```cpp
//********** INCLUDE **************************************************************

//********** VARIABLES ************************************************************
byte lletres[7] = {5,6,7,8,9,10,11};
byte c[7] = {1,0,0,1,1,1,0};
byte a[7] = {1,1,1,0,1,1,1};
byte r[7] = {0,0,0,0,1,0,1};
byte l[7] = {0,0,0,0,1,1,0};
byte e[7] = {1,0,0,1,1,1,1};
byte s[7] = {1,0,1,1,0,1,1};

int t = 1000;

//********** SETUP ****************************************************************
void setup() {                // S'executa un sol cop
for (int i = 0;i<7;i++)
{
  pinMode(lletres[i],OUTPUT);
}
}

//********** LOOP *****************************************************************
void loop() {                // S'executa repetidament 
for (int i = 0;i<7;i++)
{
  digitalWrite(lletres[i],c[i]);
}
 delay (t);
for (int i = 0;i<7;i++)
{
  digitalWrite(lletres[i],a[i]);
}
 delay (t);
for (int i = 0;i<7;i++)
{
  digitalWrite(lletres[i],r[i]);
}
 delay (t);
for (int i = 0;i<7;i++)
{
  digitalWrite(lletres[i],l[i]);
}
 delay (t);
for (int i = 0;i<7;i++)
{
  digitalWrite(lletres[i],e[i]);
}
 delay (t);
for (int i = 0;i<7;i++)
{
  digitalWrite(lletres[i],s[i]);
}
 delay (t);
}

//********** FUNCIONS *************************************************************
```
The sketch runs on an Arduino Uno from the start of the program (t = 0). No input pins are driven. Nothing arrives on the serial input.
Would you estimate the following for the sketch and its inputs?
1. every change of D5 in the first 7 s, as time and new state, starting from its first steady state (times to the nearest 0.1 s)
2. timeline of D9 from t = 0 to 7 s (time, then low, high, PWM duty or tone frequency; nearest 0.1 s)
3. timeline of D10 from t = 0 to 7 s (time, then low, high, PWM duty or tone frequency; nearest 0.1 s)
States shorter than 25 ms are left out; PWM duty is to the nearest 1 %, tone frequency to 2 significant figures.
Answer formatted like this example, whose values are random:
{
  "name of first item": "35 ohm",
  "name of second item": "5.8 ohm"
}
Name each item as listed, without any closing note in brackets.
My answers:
{
  "every change of D5 in the first 7 s, as time and new state, starting from its first steady state": "0 s high; 2 s low; 4 s high",
  "timeline of D9 from t = 0 to 7 s": "0 s high; 5 s low; 6 s high",
  "timeline of D10 from t = 0 to 7 s": "0 s high; 2 s low; 3 s high"
}
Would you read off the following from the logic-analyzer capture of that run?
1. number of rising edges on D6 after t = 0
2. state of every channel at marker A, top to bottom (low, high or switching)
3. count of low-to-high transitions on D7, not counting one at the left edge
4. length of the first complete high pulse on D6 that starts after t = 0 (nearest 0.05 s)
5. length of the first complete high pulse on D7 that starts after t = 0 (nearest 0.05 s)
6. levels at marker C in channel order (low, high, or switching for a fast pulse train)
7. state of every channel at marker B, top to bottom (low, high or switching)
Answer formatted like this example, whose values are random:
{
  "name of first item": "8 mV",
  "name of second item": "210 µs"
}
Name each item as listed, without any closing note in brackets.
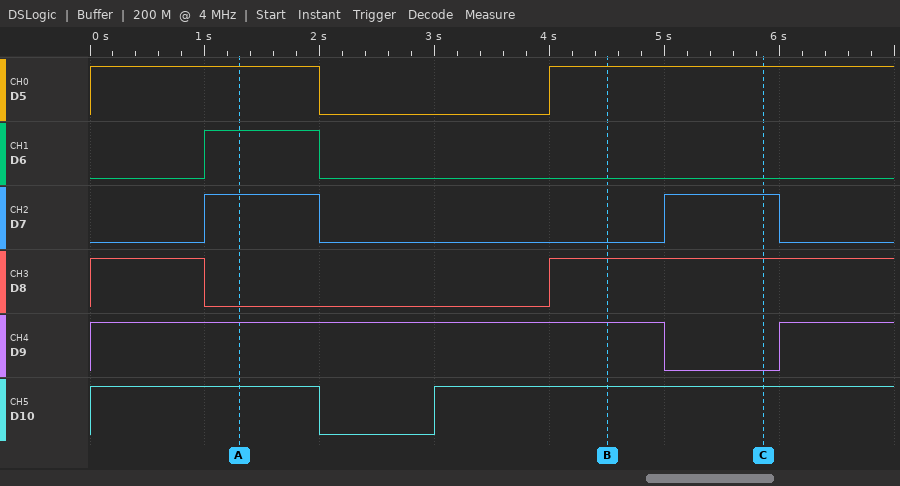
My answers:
{
  "number of rising edges on D6 after t = 0": "1",
  "state of every channel at marker A, top to bottom": "D5 high, D6 high, D7 high, D8 low, D9 high, D10 high",
  "count of low-to-high transitions on D7, not counting one at the left edge": "2",
  "length of the first complete high pulse on D6 that starts after t = 0": "1.00 s",
  "length of the first complete high pulse on D7 that starts after t = 0": "1.00 s",
  "levels at marker C in channel order": "D5 high, D6 low, D7 high, D8 high, D9 low, D10 high",
  "state of every channel at marker B, top to bottom": "D5 high, D6 low, D7 low, D8 high, D9 high, D10 high"
}
